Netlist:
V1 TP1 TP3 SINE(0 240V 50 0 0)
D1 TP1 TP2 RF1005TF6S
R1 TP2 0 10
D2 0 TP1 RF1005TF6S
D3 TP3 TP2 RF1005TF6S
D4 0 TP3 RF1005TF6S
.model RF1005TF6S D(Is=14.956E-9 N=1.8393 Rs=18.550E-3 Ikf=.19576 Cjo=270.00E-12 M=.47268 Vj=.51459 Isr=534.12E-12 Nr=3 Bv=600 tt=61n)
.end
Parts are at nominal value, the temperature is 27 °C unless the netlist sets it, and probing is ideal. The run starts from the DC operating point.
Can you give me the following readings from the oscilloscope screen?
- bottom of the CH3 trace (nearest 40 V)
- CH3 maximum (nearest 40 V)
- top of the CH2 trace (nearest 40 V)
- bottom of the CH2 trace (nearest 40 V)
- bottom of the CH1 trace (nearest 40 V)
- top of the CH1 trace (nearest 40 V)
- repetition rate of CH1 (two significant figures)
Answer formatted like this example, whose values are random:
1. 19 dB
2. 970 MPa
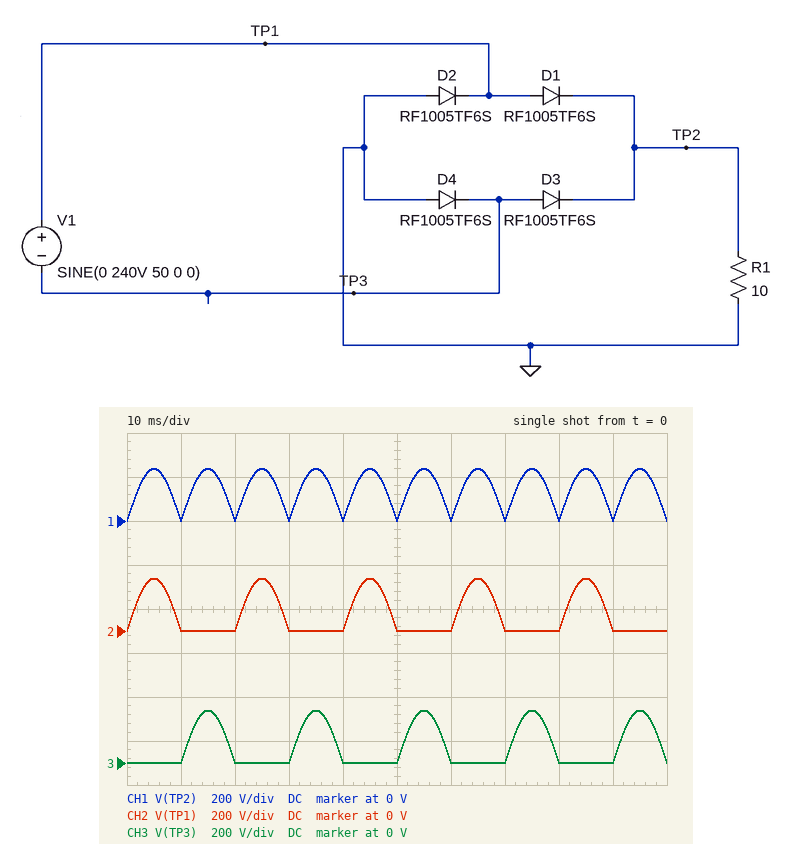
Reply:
1. 0 V
2. 240 V
3. 240 V
4. 0 V
5. 0 V
6. 240 V
7. 100 Hz
